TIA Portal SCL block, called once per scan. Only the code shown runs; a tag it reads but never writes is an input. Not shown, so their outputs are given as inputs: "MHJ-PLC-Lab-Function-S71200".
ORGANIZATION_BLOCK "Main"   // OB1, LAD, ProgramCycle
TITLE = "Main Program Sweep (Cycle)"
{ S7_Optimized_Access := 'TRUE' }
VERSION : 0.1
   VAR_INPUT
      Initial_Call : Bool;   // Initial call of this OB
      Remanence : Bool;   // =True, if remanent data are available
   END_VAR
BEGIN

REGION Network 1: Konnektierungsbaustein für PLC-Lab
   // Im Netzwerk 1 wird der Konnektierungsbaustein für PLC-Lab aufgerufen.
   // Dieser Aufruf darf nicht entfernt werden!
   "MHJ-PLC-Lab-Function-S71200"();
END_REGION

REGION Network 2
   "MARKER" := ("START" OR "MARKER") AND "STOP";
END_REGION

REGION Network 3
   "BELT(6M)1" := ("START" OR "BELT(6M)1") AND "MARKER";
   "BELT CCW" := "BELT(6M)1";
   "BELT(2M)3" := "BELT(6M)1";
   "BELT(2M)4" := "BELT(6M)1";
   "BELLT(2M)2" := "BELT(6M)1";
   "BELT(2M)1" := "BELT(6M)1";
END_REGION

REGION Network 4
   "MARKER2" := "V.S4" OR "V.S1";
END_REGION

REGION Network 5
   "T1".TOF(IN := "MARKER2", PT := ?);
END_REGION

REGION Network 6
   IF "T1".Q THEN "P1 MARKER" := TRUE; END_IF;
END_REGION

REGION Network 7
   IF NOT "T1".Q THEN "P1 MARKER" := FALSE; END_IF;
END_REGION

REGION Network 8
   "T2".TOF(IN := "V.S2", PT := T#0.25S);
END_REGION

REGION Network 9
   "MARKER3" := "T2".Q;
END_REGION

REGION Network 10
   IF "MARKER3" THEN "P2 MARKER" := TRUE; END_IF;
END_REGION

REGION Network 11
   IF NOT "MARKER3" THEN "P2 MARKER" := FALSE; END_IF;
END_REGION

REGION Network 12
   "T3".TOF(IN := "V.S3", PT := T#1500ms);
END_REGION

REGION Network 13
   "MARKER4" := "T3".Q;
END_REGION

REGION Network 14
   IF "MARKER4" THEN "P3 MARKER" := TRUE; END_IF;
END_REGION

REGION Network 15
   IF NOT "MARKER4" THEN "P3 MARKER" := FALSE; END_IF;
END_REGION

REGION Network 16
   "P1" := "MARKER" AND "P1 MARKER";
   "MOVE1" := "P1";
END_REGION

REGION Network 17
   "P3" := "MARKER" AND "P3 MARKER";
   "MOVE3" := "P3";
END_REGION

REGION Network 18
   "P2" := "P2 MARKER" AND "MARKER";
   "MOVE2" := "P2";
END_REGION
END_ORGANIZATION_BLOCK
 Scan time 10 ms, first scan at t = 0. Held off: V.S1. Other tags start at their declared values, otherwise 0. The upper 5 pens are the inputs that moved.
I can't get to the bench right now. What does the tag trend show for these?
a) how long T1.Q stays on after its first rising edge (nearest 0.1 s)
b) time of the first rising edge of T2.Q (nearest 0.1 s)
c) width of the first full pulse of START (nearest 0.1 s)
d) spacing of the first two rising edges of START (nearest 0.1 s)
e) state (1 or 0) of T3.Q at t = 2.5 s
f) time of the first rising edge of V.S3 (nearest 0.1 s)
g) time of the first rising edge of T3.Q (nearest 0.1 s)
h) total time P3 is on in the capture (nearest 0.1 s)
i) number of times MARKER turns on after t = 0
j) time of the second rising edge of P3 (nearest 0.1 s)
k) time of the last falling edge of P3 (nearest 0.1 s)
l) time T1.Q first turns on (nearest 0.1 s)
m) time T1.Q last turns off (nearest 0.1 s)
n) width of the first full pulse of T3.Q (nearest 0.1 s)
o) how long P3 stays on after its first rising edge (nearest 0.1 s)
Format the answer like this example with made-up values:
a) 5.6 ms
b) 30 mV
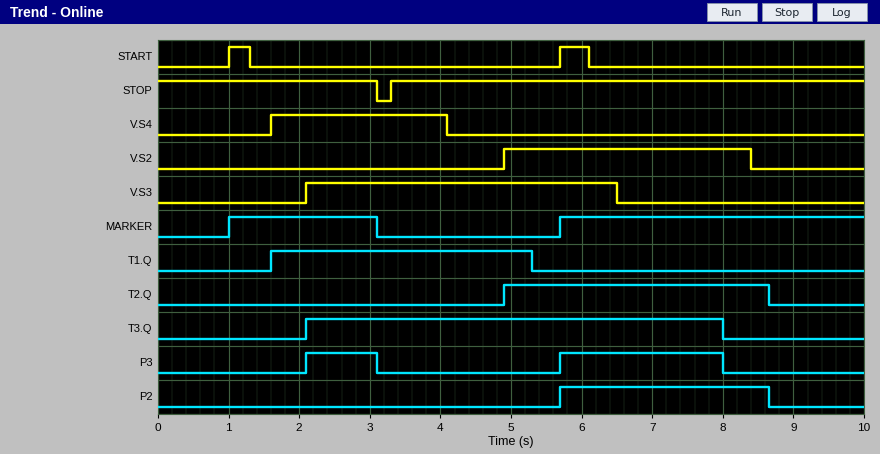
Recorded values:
a) 3.7 s
b) 4.9 s
c) 0.3 s
d) 4.7 s
e) 1
f) 2.1 s
g) 2.1 s
h) 3.3 s
i) 2
j) 5.7 s
k) 8.0 s
l) 1.6 s
m) 5.3 s
n) 5.9 s
o) 1.0 s
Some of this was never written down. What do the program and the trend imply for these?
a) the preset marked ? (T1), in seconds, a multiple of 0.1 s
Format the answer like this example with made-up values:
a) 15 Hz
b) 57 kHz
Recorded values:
a) 1.2 s
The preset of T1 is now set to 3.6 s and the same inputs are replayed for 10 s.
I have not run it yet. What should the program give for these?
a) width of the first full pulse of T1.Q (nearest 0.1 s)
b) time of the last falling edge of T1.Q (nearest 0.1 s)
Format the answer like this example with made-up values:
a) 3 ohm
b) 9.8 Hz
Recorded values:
a) 6.1 s
b) 7.7 s
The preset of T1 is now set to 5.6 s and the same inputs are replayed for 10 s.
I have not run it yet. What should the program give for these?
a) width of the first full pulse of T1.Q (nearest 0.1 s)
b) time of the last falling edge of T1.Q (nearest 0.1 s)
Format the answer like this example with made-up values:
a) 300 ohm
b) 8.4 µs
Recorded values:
a) 8.1 s
b) 9.7 s
